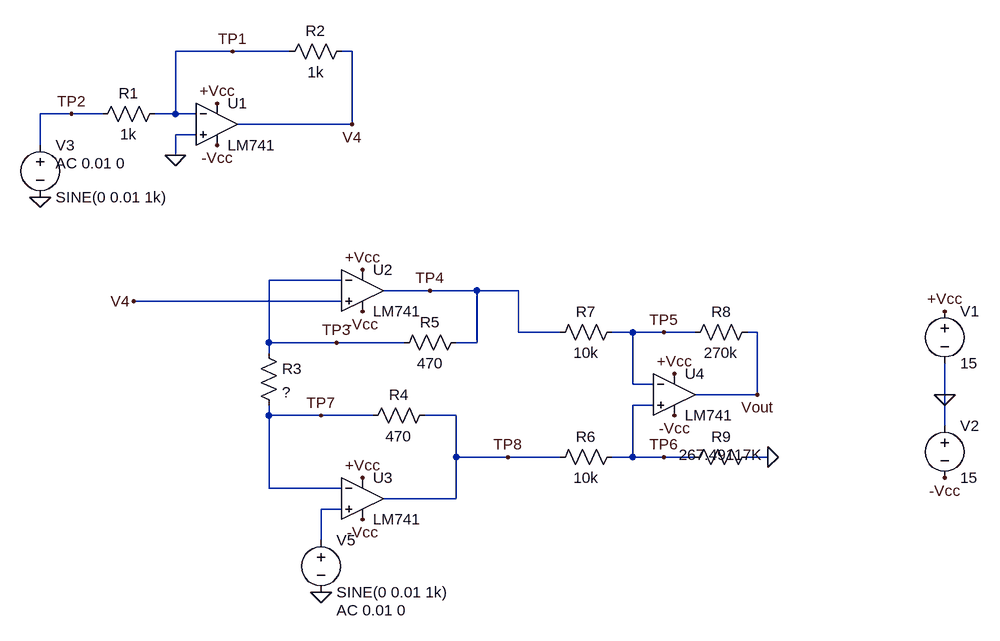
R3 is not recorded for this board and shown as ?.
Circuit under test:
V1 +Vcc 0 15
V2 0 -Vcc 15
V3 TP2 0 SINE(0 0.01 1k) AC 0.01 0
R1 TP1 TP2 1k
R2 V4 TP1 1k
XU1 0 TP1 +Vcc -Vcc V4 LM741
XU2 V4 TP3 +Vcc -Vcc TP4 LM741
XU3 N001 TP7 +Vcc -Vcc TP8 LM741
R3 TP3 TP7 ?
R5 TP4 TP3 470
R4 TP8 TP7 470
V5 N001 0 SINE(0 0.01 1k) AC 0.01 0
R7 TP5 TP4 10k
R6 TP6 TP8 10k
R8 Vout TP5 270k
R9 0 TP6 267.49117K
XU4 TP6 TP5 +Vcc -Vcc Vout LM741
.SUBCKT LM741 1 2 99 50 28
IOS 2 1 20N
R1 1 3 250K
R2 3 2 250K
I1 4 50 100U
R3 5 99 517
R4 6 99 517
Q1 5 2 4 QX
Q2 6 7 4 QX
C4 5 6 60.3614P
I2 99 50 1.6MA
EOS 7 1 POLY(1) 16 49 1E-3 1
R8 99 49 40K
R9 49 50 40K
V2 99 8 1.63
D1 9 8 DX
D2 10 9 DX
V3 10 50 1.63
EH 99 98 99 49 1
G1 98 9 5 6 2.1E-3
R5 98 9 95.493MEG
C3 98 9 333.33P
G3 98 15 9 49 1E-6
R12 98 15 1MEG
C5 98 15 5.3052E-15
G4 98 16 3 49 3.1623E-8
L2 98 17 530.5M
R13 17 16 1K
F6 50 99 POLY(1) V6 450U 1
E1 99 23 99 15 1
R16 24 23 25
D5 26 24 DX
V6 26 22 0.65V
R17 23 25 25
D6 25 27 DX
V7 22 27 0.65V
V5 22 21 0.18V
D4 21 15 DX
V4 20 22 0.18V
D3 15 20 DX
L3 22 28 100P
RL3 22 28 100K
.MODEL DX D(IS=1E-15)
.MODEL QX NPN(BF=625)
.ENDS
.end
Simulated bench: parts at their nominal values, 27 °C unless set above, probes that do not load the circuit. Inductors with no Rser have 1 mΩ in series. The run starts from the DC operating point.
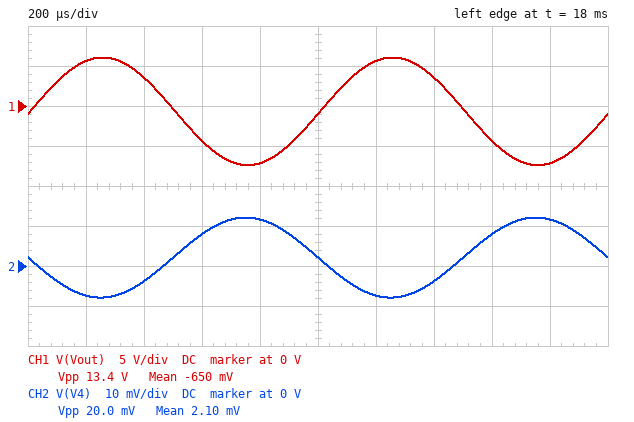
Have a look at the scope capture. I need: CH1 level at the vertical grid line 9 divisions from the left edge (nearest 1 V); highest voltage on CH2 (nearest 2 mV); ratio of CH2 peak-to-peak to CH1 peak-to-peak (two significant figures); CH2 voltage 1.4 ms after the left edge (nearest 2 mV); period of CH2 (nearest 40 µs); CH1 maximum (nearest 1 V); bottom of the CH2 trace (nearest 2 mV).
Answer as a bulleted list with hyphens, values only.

- -7 V
- 12 mV
- 0.0015
- -4 mV
- 1.00 ms
- 6 V
- -8 mV
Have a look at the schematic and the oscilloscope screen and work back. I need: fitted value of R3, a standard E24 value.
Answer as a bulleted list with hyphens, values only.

- 82 Ω
